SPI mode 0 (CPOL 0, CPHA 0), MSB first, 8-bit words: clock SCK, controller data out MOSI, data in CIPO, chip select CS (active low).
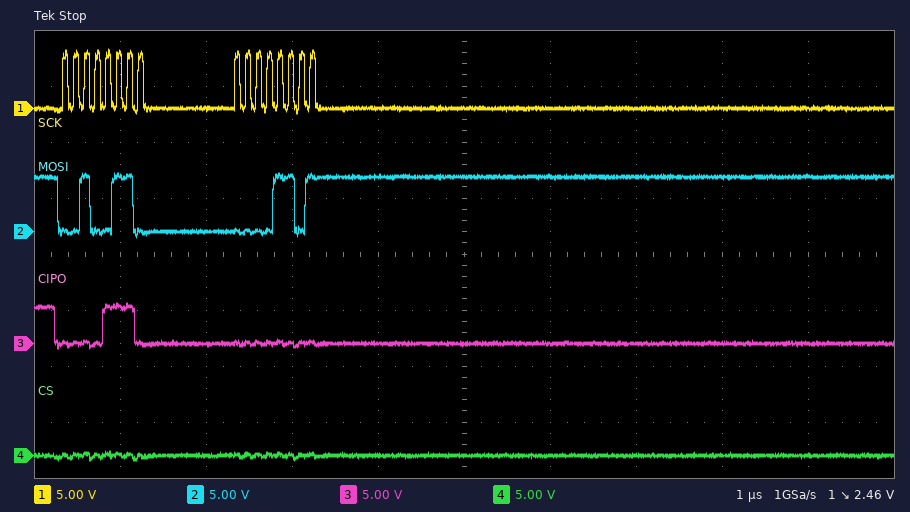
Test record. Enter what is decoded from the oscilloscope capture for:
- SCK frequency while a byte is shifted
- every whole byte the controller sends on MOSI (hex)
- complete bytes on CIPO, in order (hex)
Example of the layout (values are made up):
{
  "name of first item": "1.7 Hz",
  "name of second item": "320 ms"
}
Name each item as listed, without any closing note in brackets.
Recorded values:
{
  "SCK frequency while a byte is shifted": "8 MHz",
  "every whole byte the controller sends on MOSI": "26 0D",
  "complete bytes on CIPO, in order": "0E 00"
}
